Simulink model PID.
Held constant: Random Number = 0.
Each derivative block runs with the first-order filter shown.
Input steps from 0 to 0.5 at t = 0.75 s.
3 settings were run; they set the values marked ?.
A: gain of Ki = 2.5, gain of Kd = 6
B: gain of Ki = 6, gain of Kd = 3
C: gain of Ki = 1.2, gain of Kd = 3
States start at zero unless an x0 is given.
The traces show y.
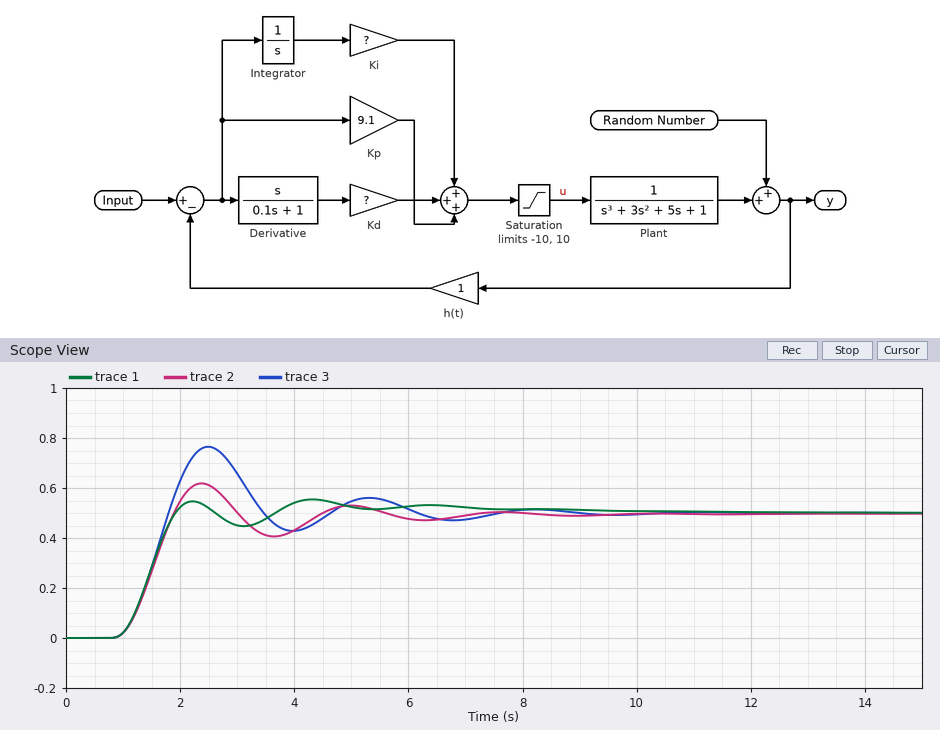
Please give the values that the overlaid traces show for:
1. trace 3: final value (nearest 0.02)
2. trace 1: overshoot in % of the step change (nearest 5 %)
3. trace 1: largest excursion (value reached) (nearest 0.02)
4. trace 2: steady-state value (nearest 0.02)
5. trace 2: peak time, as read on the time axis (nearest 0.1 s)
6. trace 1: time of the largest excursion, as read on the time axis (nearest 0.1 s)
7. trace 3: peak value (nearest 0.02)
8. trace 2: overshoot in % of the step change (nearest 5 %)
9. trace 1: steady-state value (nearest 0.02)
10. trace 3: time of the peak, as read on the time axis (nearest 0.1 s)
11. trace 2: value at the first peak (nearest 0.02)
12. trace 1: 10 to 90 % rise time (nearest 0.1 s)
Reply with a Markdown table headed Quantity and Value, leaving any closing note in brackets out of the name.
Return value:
| Quantity | Value |
|---|---|
| trace 3: final value | 0.50 |
| trace 1: overshoot in % of the step change | 10 % |
| trace 1: largest excursion (value reached) | 0.56 |
| trace 2: steady-state value | 0.50 |
| trace 2: peak time, as read on the time axis | 2.4 s |
| trace 1: time of the largest excursion, as read on the time axis | 4.3 s |
| trace 3: peak value | 0.76 |
| trace 2: overshoot in % of the step change | 25 % |
| trace 1: steady-state value | 0.50 |
| trace 3: time of the peak, as read on the time axis | 2.5 s |
| trace 2: value at the first peak | 0.62 |
| trace 1: 10 to 90 % rise time | 0.7 s |
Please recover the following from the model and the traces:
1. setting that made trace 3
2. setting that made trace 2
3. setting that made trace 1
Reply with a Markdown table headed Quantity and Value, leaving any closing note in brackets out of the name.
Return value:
| Quantity | Value |
|---|---|
| setting that made trace 3 | B |
| setting that made trace 2 | C |
| setting that made trace 1 | A |
